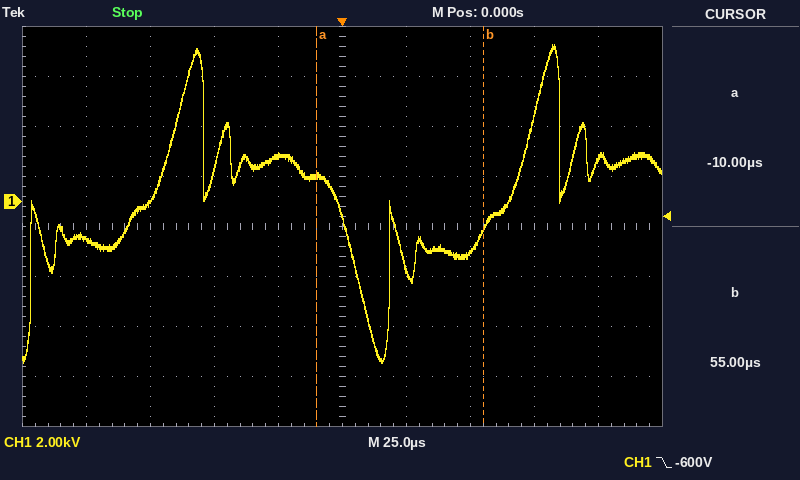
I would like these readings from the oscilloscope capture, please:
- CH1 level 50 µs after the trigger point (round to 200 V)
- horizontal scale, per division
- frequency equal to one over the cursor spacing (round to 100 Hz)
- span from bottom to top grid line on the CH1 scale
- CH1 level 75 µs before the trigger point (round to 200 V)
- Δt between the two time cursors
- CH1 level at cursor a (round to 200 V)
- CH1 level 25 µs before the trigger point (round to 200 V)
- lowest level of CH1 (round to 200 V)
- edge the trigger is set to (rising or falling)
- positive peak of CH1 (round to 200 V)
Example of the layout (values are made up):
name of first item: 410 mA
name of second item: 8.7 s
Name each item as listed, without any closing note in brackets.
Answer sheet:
CH1 level 50 µs after the trigger point: -2.0 kV
horizontal scale, per division: 25 µs
frequency equal to one over the cursor spacing: 15.4 kHz
span from bottom to top grid line on the CH1 scale: 16 kV
CH1 level 75 µs before the trigger point: 0.0 kV
Δt between the two time cursors: 65.0 µs
CH1 level at cursor a: 1.0 kV
CH1 level 25 µs before the trigger point: 1.8 kV
lowest level of CH1: -6.4 kV
edge the trigger is set to: falling
positive peak of CH1: 6.2 kV
